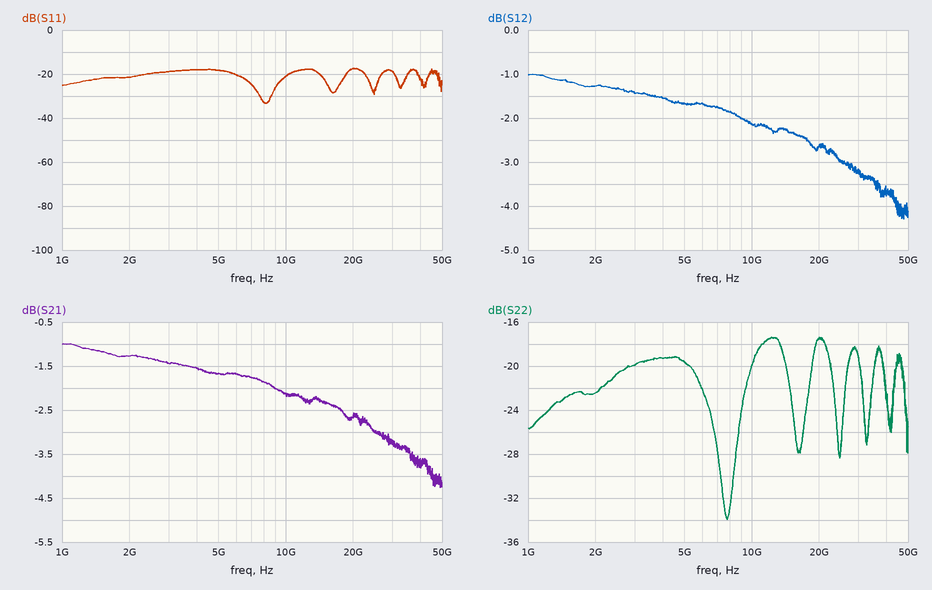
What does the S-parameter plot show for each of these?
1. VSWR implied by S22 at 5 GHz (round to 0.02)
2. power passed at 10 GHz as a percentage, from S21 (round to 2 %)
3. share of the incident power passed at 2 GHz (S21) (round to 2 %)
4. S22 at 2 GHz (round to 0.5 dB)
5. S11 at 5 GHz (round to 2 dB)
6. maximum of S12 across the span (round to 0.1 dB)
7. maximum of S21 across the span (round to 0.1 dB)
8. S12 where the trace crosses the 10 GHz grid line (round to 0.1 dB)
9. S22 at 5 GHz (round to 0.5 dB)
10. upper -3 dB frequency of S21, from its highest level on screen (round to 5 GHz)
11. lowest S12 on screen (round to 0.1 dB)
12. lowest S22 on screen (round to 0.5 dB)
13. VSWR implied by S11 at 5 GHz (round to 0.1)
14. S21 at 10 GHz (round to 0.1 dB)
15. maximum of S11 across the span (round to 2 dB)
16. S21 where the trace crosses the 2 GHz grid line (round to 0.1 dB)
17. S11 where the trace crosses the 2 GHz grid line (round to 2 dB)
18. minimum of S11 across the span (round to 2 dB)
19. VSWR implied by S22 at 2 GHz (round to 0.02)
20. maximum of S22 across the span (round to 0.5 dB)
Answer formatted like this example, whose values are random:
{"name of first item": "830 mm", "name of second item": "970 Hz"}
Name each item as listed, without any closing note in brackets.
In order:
{"VSWR implied by S22 at 5 GHz": "1.24", "power passed at 10 GHz as a percentage, from S21": "62 %", "share of the incident power passed at 2 GHz (S21)": "74 %", "S22 at 2 GHz": "-22.5 dB", "S11 at 5 GHz": "-18 dB", "maximum of S12 across the span": "-1.0 dB", "maximum of S21 across the span": "-1.0 dB", "S12 where the trace crosses the 10 GHz grid line": "-2.1 dB", "S22 at 5 GHz": "-19.5 dB", "upper -3 dB frequency of S21, from its highest level on screen": "45 GHz", "lowest S12 on screen": "-4.3 dB", "lowest S22 on screen": "-34.0 dB", "VSWR implied by S11 at 5 GHz": "1.3", "S21 at 10 GHz": "-2.1 dB", "maximum of S11 across the span": "-18 dB", "S21 where the trace crosses the 2 GHz grid line": "-1.3 dB", "S11 where the trace crosses the 2 GHz grid line": "-22 dB", "minimum of S11 across the span": "-34 dB", "VSWR implied by S22 at 2 GHz": "1.16", "maximum of S22 across the span": "-17.5 dB"}
